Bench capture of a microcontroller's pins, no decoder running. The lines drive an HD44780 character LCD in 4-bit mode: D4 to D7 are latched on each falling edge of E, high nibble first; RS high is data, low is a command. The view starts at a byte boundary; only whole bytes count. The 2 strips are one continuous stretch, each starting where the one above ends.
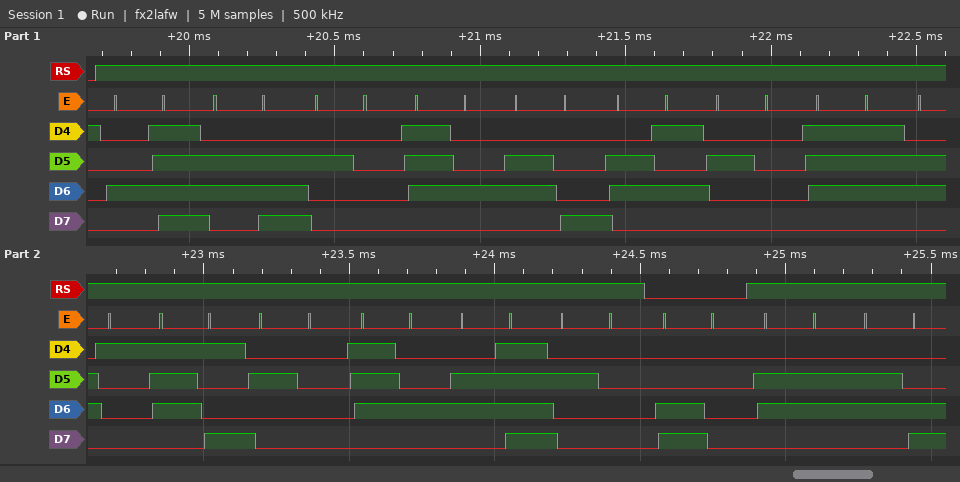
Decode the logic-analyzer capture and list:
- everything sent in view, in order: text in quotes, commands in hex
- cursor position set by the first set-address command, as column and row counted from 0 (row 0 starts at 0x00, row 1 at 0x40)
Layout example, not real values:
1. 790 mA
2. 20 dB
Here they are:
1. "On the way to " 0xC0 "fl"
2. column 0, row 1
